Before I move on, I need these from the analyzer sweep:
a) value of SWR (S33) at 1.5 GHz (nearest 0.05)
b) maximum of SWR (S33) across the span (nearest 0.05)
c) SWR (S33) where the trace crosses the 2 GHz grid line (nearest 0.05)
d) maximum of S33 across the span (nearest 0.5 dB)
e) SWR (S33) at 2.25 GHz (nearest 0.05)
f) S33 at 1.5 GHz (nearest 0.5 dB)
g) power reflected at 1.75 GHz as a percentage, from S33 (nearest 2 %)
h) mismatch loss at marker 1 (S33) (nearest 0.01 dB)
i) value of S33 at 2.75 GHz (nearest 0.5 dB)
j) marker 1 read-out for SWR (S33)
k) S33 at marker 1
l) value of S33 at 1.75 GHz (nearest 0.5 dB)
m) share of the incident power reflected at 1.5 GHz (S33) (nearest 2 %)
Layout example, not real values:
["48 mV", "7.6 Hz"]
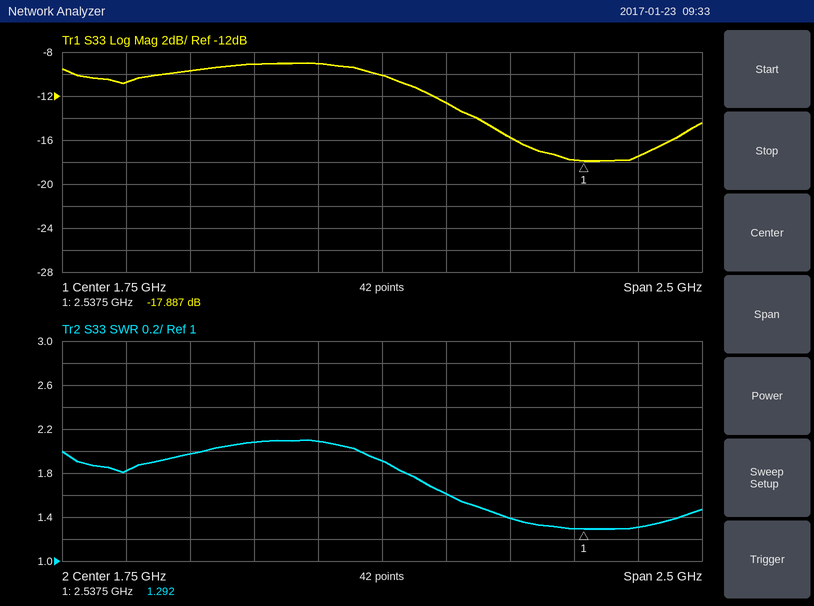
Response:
["2.10", "2.10", "1.60", "-9.0 dB", "1.40", "-9.0 dB", "10 %", "0.07 dB", "-17.5 dB", "1.292", "-17.887 dB", "-10.0 dB", "12 %"]
